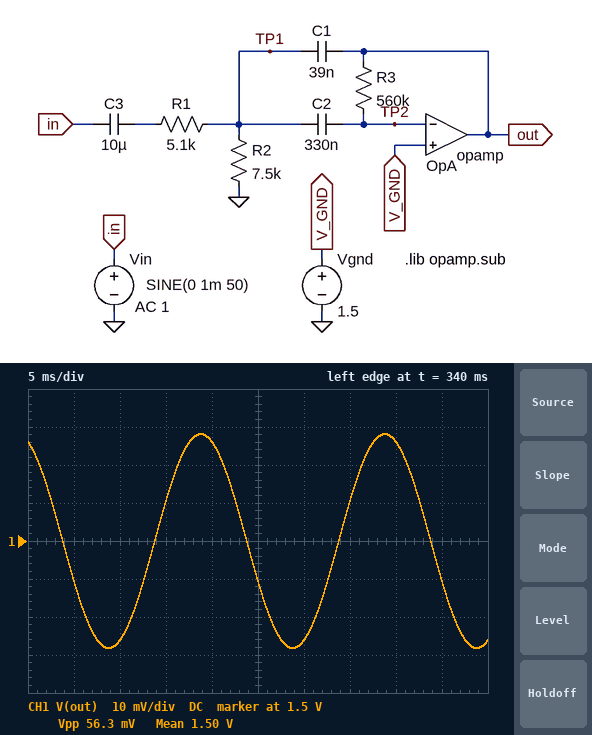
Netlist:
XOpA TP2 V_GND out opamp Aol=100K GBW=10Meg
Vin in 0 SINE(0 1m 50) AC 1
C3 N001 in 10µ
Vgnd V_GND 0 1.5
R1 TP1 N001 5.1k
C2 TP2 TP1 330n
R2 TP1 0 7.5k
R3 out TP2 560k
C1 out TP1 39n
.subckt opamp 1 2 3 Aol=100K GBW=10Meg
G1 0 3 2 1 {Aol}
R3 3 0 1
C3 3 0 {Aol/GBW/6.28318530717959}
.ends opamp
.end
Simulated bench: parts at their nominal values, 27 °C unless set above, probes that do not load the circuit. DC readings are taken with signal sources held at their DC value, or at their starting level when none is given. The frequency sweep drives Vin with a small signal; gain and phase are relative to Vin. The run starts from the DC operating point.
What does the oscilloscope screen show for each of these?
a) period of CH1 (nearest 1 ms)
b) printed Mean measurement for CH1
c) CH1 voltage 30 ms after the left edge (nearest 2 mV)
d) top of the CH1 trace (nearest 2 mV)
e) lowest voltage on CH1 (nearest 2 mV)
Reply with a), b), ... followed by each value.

a) 20 ms
b) 1.50 V
c) 1.474 V
d) 1.528 V
e) 1.472 V
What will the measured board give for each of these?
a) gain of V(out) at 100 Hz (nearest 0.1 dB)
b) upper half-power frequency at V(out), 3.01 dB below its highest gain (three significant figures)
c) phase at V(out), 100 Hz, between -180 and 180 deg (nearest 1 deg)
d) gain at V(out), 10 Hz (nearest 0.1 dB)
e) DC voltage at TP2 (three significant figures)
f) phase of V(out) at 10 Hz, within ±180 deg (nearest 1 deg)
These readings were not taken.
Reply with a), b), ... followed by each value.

a) 19.1 dB
b) 39.6 Hz
c) 97 deg
d) 17.4 dB
e) 1.50 V
f) -88 deg
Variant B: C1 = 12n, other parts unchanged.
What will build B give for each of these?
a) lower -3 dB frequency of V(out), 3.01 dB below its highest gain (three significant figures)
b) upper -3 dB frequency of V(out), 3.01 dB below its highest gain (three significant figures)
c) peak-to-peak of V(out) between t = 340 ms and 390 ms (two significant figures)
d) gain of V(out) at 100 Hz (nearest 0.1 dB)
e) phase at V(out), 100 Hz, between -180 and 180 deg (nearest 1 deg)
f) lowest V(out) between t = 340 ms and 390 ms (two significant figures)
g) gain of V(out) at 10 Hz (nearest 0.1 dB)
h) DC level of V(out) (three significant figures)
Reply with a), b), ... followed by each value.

a) 49.9 Hz
b) 76.3 Hz
c) 140 mV
d) 31.7 dB
e) 114 deg
f) 1.4 V
g) 16.8 dB
h) 1.50 V
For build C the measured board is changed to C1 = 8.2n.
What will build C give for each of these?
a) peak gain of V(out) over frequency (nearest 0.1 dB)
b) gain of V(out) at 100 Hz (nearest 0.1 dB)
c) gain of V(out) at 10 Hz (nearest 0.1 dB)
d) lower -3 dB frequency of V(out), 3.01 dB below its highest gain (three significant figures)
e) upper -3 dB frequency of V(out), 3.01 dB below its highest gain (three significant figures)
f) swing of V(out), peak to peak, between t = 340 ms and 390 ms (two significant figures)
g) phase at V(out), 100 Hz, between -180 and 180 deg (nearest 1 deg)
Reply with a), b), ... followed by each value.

a) 40.1 dB
b) 36.3 dB
c) 16.8 dB
d) 58.2 Hz
e) 95.6 Hz
f) 110 mV
g) 131 deg
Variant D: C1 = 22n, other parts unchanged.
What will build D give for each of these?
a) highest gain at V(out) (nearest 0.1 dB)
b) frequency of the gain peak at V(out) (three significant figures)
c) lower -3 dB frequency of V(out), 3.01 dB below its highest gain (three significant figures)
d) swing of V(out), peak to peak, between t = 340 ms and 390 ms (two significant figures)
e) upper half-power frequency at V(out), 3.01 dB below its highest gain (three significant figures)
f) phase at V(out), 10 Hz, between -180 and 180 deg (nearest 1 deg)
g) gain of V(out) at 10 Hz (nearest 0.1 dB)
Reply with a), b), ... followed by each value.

a) 39.1 dB
b) 45.6 Hz
c) 38.4 Hz
d) 160 mV
e) 54.1 Hz
f) -87 deg
g) 17.0 dB
